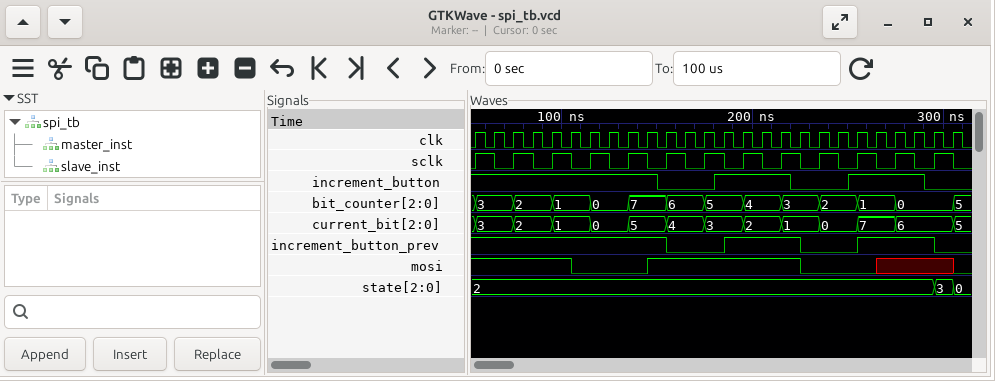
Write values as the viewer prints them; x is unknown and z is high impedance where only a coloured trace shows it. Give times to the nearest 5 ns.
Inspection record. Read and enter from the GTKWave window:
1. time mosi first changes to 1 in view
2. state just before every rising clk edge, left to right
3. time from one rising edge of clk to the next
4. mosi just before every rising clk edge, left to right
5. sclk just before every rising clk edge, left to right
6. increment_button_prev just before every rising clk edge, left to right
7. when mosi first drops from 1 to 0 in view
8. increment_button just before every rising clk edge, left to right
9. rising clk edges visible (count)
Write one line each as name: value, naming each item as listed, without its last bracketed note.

time mosi first changes to 1 in view: 145 ns
state just before every rising clk edge, left to right: 2, 2, 2, 2, 2, 2, 2, 2, 2, 2, 2, 2, 2, 2, 2, 2, 2, 2, 2, 2, 2, 2, 2, 2, 2, 3
time from one rising edge of clk to the next: 10 ns
mosi just before every rising clk edge, left to right: 1 1 1 1 1 1 0 0 0 0 1 1 1 1 1 1 1 1 0 0 0 0 x x x x
sclk just before every rising clk edge, left to right: 0 1 0 1 0 1 0 1 0 1 0 1 0 1 0 1 0 1 0 1 0 1 0 1 0 1
increment_button_prev just before every rising clk edge, left to right: 1 1 1 1 1 1 1 1 1 1 1 0 0 0 1 1 1 1 0 0 0 1 1 1 1 0
when mosi first drops from 1 to 0 in view: 105 ns
increment_button just before every rising clk edge, left to right: 1 1 1 1 1 1 1 1 1 1 0 0 0 1 1 1 1 0 0 0 1 1 1 1 0 0
rising clk edges visible: 26
